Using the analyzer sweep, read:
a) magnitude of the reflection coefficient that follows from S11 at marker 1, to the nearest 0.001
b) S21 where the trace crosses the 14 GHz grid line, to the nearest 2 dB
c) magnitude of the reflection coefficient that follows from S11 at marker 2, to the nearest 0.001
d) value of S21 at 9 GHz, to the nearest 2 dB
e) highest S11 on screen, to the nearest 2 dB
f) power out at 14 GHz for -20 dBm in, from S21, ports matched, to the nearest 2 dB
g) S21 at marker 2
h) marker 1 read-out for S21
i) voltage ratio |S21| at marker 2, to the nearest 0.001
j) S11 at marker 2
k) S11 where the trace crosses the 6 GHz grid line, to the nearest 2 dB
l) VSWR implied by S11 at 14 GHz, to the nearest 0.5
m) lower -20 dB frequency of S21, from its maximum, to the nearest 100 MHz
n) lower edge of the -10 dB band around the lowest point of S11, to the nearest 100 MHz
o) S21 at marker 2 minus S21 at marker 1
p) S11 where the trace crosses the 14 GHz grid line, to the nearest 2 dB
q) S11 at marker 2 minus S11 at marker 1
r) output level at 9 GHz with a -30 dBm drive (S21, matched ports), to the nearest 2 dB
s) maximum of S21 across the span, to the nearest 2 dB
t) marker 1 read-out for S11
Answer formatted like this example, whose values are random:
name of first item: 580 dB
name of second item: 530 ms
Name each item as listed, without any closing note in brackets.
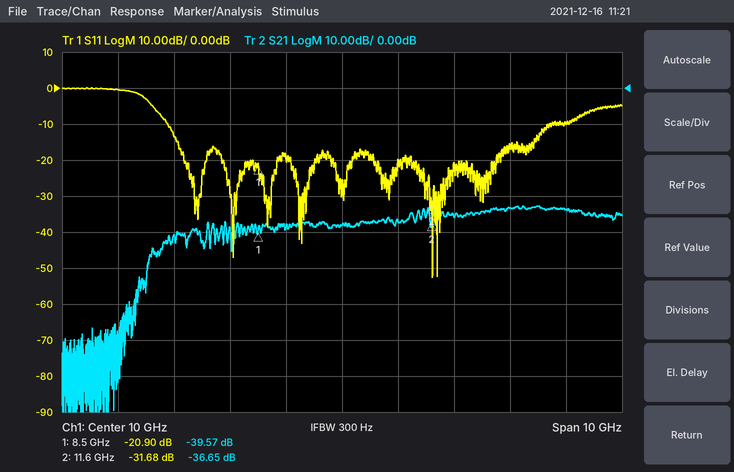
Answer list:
magnitude of the reflection coefficient that follows from S11 at marker 1, to the nearest 0.001: 0.090
S21 where the trace crosses the 14 GHz grid line, to the nearest 2 dB: -34 dB
magnitude of the reflection coefficient that follows from S11 at marker 2, to the nearest 0.001: 0.026
value of S21 at 9 GHz, to the nearest 2 dB: -38 dB
highest S11 on screen, to the nearest 2 dB: 0 dB
power out at 14 GHz for -20 dBm in, from S21, ports matched, to the nearest 2 dB: -54 dBm
S21 at marker 2: -36.65 dB
marker 1 read-out for S21: -39.57 dB
voltage ratio |S21| at marker 2, to the nearest 0.001: 0.015
S11 at marker 2: -31.68 dB
S11 where the trace crosses the 6 GHz grid line, to the nearest 2 dB: 0 dB
VSWR implied by S11 at 14 GHz, to the nearest 0.5: 2.0
lower -20 dB frequency of S21, from its maximum, to the nearest 100 MHz: 6.5 GHz
lower edge of the -10 dB band around the lowest point of S11, to the nearest 100 MHz: 6.9 GHz
S21 at marker 2 minus S21 at marker 1: 2.92 dB
S11 where the trace crosses the 14 GHz grid line, to the nearest 2 dB: -10 dB
S11 at marker 2 minus S11 at marker 1: -10.78 dB
output level at 9 GHz with a -30 dBm drive (S21, matched ports), to the nearest 2 dB: -68 dBm
maximum of S21 across the span, to the nearest 2 dB: -32 dB
marker 1 read-out for S11: -20.90 dB
